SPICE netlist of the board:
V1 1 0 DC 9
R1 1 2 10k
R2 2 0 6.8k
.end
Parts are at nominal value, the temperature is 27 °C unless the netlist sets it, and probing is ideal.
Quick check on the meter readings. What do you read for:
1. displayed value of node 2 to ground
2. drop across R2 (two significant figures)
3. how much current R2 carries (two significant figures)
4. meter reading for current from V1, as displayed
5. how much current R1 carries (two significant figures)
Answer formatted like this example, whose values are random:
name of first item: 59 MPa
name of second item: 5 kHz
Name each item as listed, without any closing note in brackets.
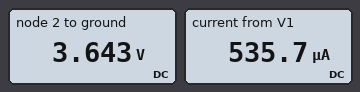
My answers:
displayed value of node 2 to ground: 3.643 V
drop across R2: 3.6 V
how much current R2 carries: 540 µA
meter reading for current from V1, as displayed: 535.7 µA
how much current R1 carries: 540 µA
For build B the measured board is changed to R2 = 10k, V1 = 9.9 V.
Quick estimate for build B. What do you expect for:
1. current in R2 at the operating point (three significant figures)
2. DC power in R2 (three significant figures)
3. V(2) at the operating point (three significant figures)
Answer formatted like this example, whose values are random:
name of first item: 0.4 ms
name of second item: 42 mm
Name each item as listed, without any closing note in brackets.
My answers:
current in R2 at the operating point: 495 µA
DC power in R2: 2.45 mW
V(2) at the operating point: 4.95 V
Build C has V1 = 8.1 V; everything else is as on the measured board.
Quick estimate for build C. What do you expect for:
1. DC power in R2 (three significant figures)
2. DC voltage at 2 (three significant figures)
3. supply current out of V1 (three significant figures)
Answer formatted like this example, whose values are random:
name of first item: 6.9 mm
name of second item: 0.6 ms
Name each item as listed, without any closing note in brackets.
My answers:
DC power in R2: 1.58 mW
DC voltage at 2: 3.28 V
supply current out of V1: 482 µA
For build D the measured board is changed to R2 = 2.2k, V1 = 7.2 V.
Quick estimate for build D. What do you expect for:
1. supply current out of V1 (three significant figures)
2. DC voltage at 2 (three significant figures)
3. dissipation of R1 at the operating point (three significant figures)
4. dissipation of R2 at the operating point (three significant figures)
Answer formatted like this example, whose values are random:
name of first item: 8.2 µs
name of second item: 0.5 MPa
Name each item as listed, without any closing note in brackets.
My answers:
supply current out of V1: 590 µA
DC voltage at 2: 1.30 V
dissipation of R1 at the operating point: 3.48 mW
dissipation of R2 at the operating point: 766 µW
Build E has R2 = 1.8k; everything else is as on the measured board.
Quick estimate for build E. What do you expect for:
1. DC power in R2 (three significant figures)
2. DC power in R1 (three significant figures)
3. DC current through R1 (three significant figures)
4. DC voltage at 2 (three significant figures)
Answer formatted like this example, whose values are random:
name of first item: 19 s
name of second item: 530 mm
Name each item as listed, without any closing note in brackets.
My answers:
DC power in R2: 1.05 mW
DC power in R1: 5.82 mW
DC current through R1: 763 µA
DC voltage at 2: 1.37 V
